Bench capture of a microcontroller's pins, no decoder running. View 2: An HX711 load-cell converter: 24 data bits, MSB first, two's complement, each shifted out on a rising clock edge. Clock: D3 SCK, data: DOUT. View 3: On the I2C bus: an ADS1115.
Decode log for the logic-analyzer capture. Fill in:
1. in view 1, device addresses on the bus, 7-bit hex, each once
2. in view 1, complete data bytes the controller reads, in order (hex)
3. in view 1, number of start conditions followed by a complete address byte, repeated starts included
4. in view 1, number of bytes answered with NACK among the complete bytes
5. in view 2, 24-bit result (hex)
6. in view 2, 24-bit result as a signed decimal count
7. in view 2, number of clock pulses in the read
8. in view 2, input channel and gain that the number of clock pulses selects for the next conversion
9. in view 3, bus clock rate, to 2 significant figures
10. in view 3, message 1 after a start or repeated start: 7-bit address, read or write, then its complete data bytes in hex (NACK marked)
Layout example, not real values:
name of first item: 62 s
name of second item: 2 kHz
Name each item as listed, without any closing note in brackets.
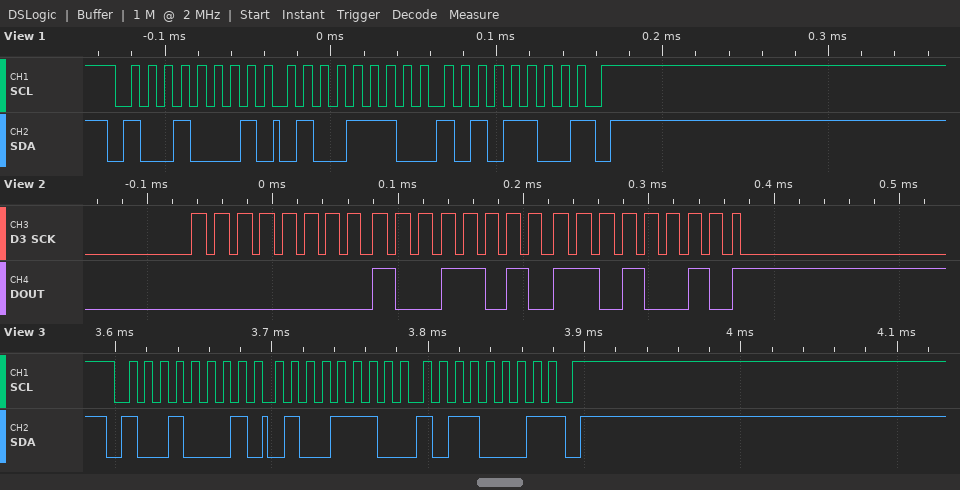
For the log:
in view 1, device addresses on the bus, 7-bit hex, each once: 0x48
in view 1, complete data bytes the controller reads, in order: 4E AC
in view 1, number of start conditions followed by a complete address byte, repeated starts included: 1
in view 1, number of bytes answered with NACK among the complete bytes: 1
in view 2, 24-bit result: 0x009AD2
in view 2, 24-bit result as a signed decimal count: 39634
in view 2, number of clock pulses in the read: 25
in view 2, input channel and gain that the number of clock pulses selects for the next conversion: channel A, gain 128
in view 3, bus clock rate, to 2 significant figures: 100 kHz
in view 3, message 1 after a start or repeated start: 7-bit address, read or write, then its complete data bytes in hex: 0x48 read: 4E B1 NACK
